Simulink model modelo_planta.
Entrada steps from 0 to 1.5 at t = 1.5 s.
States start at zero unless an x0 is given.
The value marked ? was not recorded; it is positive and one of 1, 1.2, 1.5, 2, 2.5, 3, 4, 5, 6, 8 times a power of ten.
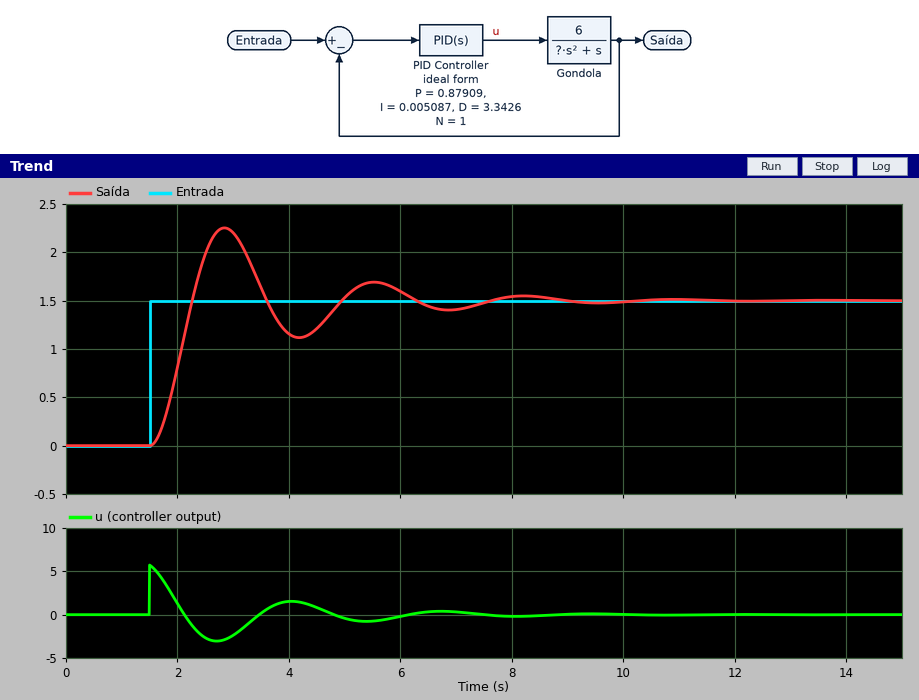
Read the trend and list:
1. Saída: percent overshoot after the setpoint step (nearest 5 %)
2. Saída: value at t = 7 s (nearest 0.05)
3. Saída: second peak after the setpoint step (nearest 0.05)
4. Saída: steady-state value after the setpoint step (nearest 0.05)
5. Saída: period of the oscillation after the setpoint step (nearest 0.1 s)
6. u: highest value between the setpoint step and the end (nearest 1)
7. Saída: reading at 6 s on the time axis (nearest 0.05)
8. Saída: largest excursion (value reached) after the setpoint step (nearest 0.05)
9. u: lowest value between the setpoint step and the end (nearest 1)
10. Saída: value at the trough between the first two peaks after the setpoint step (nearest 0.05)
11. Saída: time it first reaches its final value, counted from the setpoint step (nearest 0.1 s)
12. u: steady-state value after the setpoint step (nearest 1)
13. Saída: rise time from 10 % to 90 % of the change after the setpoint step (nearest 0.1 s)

50 %
1.40
1.70
1.50
2.7 s
6
1.60
2.25
-3
1.10
0.8 s
0
0.5 s
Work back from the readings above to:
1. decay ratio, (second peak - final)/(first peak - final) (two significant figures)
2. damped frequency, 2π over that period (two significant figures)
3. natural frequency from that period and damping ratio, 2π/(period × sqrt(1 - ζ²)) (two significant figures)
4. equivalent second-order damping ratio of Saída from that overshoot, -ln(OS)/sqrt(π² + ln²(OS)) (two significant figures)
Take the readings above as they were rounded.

0.27
2.3 rad/s
2.4 rad/s
0.22
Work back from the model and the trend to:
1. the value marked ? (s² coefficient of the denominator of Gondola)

4
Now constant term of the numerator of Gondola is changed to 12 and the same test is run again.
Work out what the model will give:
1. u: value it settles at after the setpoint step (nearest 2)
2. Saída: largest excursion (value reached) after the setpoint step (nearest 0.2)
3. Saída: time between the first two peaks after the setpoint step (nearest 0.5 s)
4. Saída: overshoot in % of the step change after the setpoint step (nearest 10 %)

0
2.4
2.0 s
60 %
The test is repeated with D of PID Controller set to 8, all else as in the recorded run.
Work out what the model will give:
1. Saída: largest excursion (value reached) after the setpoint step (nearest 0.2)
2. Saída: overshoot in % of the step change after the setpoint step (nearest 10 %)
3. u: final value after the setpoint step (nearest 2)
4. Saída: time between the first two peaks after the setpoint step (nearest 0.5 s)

2.4
60 %
0
2.0 s
